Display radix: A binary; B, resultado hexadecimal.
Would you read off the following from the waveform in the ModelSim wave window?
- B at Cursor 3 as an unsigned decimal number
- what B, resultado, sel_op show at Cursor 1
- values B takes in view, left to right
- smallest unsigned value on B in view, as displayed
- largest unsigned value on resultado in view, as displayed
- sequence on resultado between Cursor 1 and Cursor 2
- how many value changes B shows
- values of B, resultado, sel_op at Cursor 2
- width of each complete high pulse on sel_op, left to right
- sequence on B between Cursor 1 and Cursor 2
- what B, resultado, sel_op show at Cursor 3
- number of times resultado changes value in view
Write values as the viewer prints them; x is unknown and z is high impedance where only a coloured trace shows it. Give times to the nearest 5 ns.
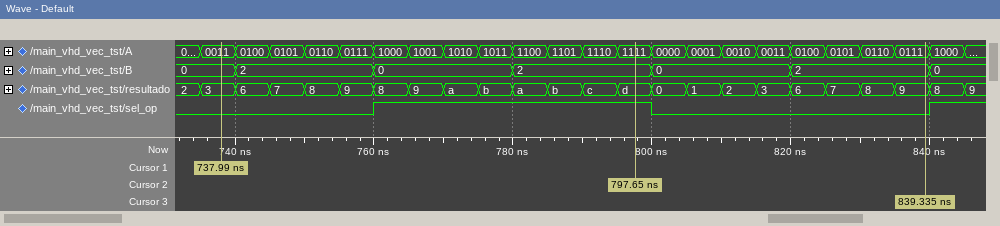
2
B=0, resultado=3, sel_op=0
0, 2, 0, 2, 0, 2, 0
0
d
3, 6, 7, 8, 9, 8, 9, a, b, a, b, c, d
6
B=2, resultado=d, sel_op=1
40 ns
0, 2, 0, 2
B=2, resultado=9, sel_op=0
23
